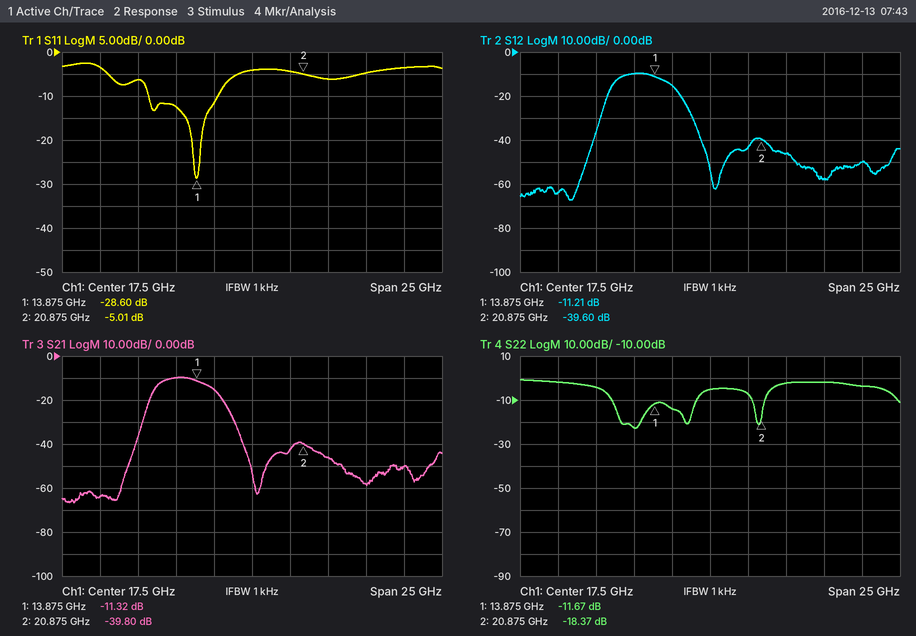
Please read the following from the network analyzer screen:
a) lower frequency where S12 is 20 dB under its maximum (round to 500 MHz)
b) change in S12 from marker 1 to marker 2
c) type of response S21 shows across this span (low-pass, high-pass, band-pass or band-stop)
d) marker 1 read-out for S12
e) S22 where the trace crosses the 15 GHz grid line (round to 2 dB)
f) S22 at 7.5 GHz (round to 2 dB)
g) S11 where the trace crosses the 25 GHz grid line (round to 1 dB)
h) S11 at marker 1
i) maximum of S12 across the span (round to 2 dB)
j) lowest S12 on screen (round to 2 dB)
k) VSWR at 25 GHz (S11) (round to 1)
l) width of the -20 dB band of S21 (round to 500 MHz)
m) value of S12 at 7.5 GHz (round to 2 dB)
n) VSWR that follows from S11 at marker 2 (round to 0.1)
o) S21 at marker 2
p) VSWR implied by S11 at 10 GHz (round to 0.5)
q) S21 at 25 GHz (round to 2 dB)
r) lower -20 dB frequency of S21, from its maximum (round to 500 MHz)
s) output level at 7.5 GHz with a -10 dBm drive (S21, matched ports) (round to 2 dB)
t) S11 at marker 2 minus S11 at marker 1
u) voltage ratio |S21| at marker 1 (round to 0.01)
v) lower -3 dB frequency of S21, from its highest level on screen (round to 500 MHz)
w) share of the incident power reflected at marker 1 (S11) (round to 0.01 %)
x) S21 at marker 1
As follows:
10.5 GHz
-28.39 dB
band-pass
-11.21 dB
-14 dB
-2 dB
-5 dB
-28.60 dB
-10 dB
-68 dB
4
6.0 GHz
-64 dB
3.6
-39.80 dB
3.0
-58 dB
10.5 GHz
-74 dBm
23.59 dB
0.27
11.5 GHz
0.14 %
-11.32 dB
